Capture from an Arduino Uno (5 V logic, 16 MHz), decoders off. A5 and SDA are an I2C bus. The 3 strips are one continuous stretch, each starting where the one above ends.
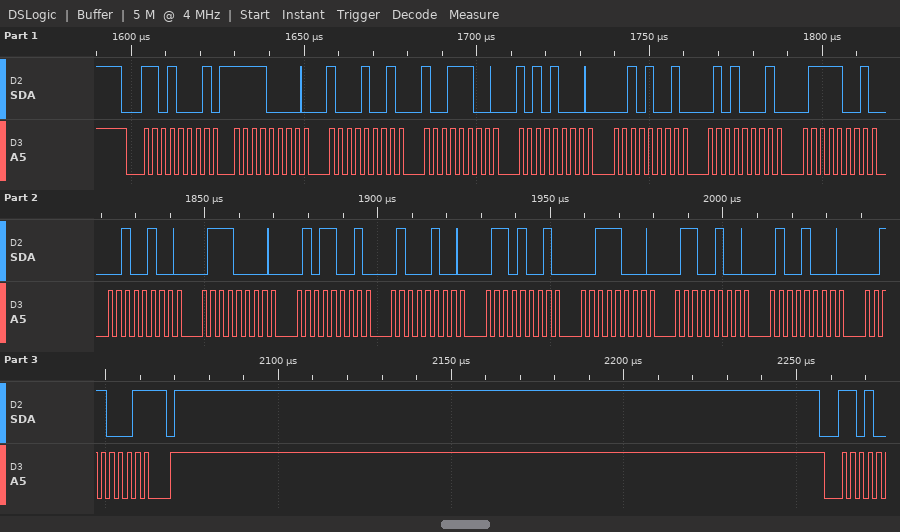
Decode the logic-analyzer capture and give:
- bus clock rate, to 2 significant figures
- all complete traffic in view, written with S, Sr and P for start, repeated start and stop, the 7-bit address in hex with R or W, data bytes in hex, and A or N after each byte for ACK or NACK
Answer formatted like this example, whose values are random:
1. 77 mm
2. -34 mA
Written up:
1. 400 kHz
2. S 68R A F0 A 89 A 9C A A8 A 29 A 51 A 79 A 24 A 70 A 59 A 44 A 69 A 38 A 64 A 48 A 31 N P
